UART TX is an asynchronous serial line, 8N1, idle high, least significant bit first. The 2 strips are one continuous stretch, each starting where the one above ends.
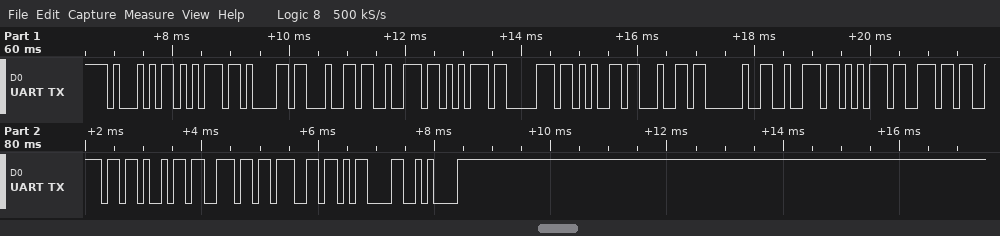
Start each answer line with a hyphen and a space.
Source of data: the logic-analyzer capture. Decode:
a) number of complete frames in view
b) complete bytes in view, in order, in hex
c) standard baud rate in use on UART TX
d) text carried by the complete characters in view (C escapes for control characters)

- 19
- 51 75 61 64 72 75 70 65 64 20 72 75 6E 6E 69 6E 67 0D 0A
- 9600 baud
- "Quadruped running\r\n"
